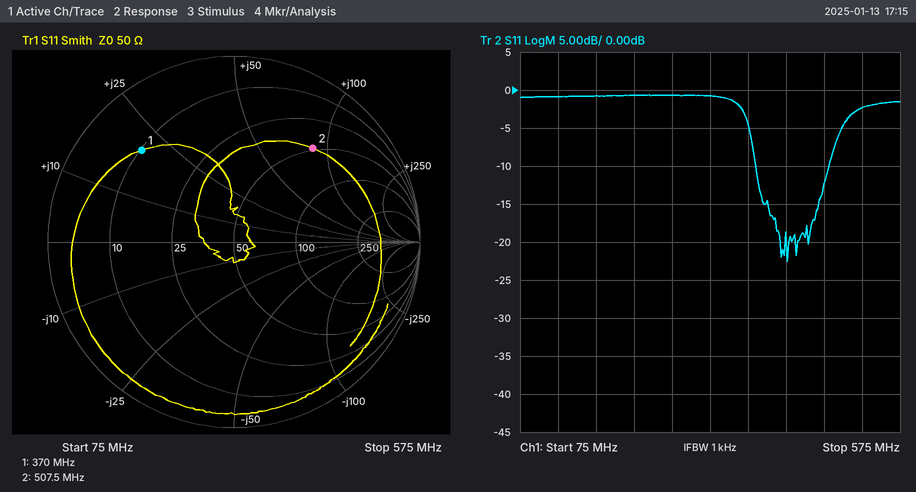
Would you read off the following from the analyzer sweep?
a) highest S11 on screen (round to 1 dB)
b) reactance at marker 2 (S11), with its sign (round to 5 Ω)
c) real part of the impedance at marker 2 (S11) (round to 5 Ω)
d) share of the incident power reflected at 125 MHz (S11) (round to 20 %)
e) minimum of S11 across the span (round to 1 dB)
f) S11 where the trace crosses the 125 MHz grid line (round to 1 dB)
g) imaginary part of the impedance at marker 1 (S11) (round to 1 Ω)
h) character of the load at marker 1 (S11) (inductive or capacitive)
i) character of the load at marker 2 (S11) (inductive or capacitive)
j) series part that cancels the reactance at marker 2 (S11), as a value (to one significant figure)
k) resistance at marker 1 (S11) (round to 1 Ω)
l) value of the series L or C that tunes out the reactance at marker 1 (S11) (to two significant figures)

-1 dB
+85 Ω
50 Ω
80 %
-23 dB
-1 dB
+20 Ω
inductive
inductive
4 pF
10 Ω
22 pF
